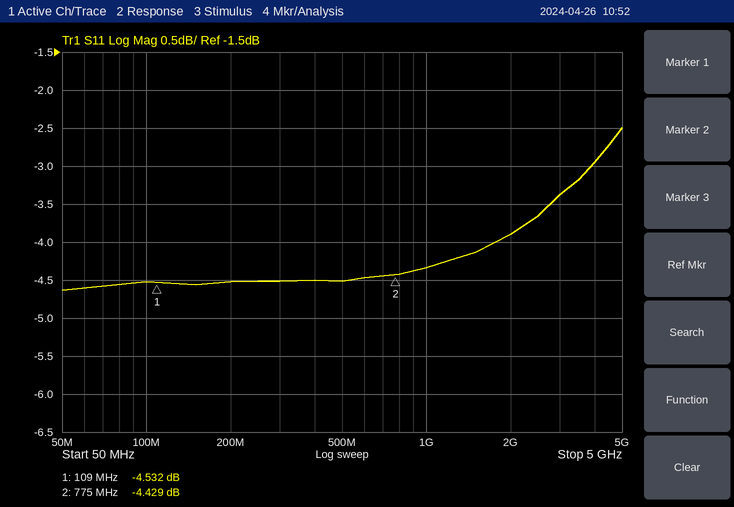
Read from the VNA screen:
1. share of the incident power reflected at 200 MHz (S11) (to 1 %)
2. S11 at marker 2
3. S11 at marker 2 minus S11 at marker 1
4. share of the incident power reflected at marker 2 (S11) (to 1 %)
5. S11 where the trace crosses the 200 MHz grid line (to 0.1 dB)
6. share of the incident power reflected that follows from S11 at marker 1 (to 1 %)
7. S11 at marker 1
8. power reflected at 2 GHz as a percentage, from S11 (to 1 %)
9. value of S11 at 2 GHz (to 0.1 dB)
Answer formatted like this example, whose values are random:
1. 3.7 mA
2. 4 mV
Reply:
1. 35 %
2. -4.429 dB
3. 0.103 dB
4. 36 %
5. -4.5 dB
6. 35 %
7. -4.532 dB
8. 41 %
9. -3.9 dB
